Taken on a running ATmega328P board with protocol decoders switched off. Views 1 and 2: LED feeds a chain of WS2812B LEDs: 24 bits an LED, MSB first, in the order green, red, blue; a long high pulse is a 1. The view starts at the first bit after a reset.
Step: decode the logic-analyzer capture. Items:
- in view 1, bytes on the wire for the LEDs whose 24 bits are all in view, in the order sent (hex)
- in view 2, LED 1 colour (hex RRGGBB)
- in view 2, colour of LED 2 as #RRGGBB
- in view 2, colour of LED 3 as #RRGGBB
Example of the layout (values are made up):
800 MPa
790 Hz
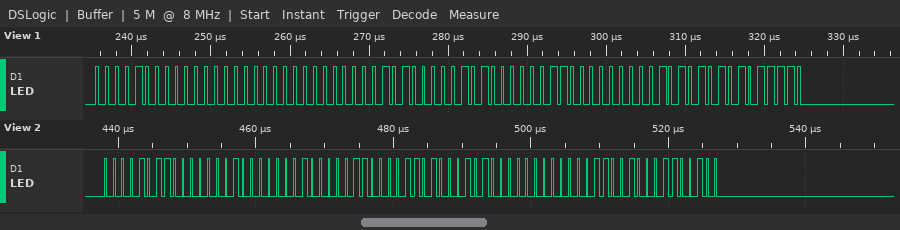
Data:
08 00 00 05 05 03 00 55 5E
#010B01
#1A0628
#640064
